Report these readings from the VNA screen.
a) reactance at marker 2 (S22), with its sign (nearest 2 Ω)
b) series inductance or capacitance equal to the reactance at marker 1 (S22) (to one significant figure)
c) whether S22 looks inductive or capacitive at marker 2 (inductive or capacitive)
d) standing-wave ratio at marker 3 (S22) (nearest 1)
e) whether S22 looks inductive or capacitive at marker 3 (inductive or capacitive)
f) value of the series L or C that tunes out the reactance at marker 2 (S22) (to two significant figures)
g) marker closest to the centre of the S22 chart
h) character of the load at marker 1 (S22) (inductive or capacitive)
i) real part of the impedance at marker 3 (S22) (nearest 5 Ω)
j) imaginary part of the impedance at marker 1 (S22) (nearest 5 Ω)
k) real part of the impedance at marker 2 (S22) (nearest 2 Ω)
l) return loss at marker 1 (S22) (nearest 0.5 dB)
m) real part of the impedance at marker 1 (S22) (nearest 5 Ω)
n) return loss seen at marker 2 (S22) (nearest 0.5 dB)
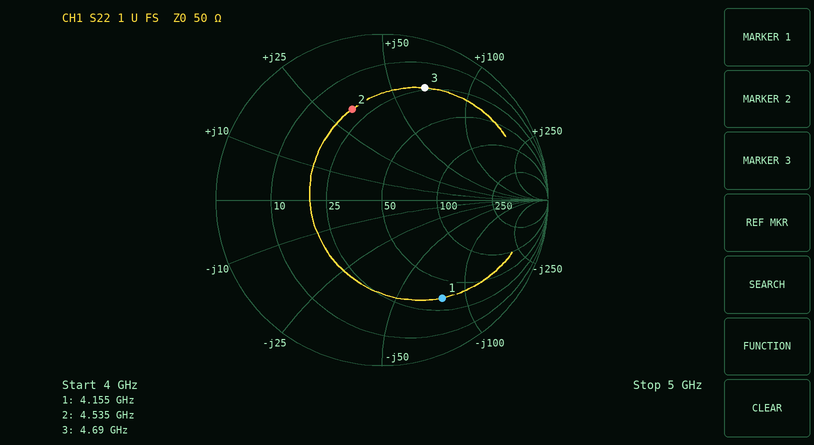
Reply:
+32 Ω
500 fF
inductive
6
inductive
1.1 pF
marker 2
capacitive
25 Ω
-80 Ω
20 Ω
3.0 dB
35 Ω
5.0 dB
